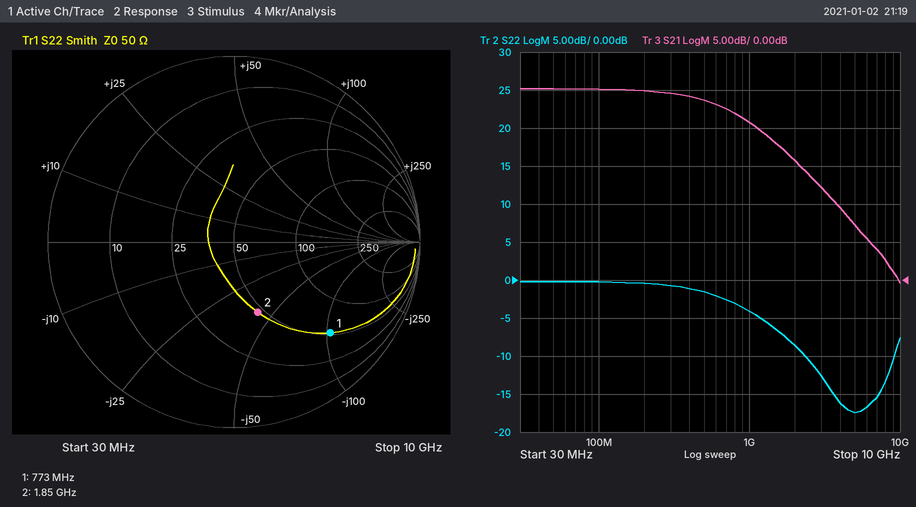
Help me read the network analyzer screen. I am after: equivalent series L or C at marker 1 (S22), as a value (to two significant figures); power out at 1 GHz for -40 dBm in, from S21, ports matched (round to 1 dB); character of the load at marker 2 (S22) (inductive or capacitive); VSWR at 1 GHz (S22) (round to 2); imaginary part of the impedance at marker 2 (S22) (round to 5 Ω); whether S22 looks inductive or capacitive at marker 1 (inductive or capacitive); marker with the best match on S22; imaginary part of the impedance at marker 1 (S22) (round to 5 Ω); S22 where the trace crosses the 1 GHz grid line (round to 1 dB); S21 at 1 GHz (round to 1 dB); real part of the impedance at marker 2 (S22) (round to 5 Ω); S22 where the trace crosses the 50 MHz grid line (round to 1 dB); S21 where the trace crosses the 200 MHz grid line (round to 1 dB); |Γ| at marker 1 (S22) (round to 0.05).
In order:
2.0 pF
-19 dBm
capacitive
4
-40 Ω
capacitive
marker 2
-105 Ω
-4 dB
21 dB
45 Ω
0 dB
25 dB
0.70
